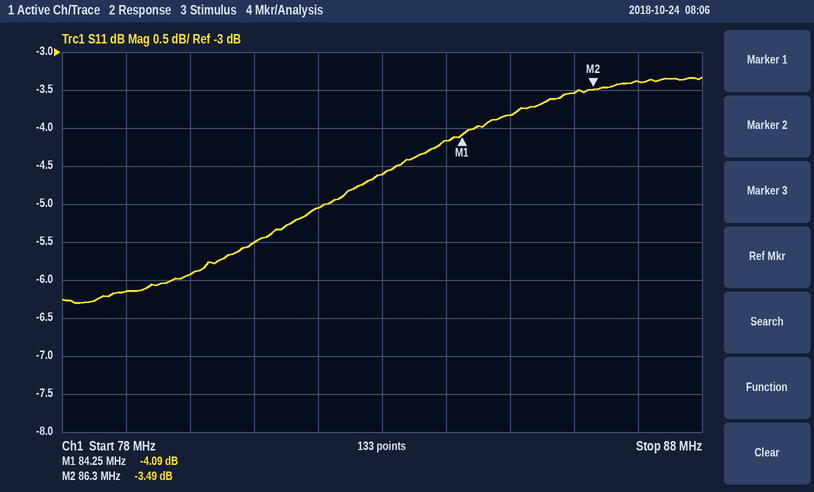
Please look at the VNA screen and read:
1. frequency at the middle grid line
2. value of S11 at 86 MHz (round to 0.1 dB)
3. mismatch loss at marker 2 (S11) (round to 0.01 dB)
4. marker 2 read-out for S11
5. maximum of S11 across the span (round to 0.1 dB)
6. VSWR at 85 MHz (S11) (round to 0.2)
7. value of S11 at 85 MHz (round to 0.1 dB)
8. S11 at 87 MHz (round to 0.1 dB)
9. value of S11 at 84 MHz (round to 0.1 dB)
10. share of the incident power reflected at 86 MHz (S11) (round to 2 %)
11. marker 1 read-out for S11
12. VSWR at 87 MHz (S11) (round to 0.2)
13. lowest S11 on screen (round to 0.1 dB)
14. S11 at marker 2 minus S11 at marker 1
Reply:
83 MHz
-3.5 dB
2.58 dB
-3.49 dB
-3.3 dB
4.6
-3.8 dB
-3.4 dB
-4.2 dB
44 %
-4.09 dB
5.2
-6.3 dB
0.60 dB
